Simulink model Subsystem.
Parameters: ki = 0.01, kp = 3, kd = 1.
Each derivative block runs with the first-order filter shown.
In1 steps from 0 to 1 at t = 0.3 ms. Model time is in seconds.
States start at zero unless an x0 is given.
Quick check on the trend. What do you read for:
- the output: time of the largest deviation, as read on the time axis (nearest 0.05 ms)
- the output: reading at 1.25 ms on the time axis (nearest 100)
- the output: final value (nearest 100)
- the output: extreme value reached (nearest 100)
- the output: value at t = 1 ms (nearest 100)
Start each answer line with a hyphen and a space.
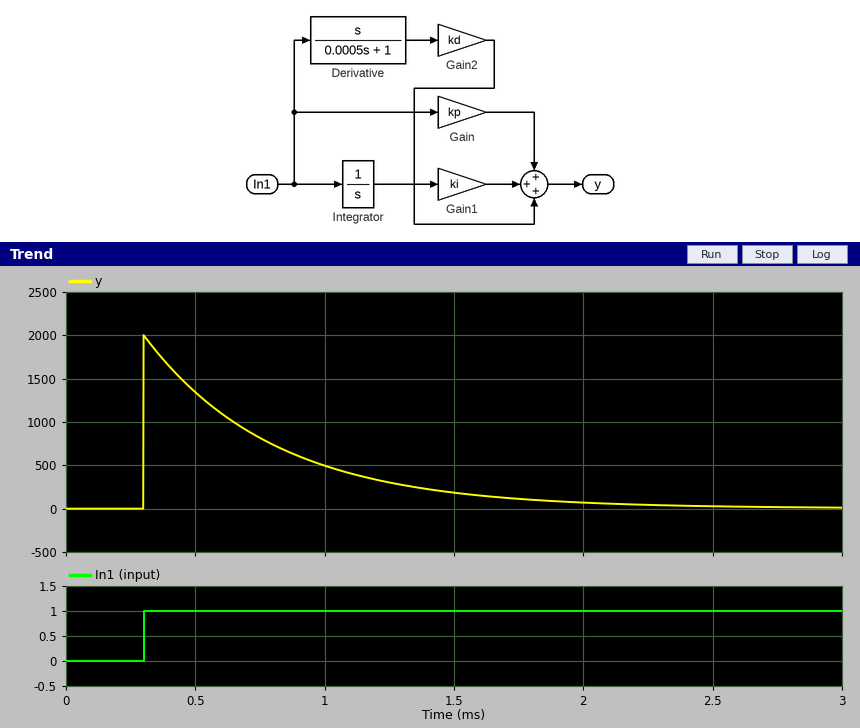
- 0.30 ms
- 300
- 0
- 2000
- 500
